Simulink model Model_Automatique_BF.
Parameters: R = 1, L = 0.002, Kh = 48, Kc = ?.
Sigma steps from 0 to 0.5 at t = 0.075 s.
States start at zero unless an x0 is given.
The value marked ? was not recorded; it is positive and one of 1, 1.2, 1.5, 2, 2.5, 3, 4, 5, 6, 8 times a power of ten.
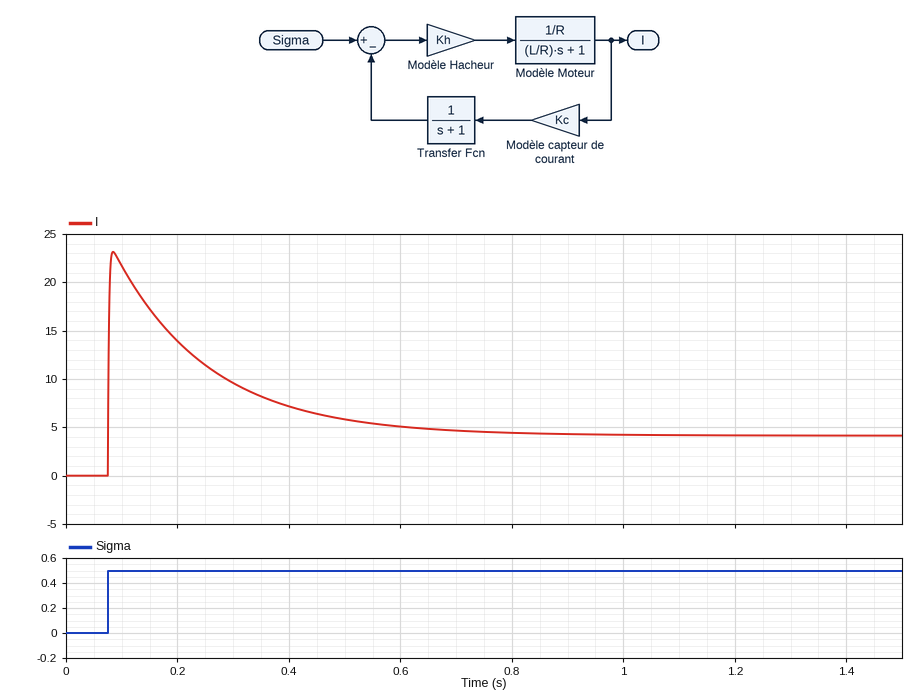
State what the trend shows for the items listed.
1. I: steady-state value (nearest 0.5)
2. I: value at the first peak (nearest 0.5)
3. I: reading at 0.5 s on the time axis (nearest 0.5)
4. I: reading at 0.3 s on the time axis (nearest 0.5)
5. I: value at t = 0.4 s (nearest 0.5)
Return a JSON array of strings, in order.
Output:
["4.0", "23.0", "6.0", "9.5", "7.0"]
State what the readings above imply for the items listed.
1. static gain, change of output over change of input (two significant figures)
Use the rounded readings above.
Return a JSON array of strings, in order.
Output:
["8.0"]
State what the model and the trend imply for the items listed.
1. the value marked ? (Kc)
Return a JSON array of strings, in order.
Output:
["0.1"]
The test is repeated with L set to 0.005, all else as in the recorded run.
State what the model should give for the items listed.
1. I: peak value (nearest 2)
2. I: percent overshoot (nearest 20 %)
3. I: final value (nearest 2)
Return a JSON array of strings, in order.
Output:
["22", "440 %", "4"]
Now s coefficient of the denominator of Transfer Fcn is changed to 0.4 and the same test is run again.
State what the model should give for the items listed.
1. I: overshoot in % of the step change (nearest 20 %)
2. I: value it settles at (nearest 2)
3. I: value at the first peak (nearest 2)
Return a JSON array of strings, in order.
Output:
["440 %", "4", "22"]
